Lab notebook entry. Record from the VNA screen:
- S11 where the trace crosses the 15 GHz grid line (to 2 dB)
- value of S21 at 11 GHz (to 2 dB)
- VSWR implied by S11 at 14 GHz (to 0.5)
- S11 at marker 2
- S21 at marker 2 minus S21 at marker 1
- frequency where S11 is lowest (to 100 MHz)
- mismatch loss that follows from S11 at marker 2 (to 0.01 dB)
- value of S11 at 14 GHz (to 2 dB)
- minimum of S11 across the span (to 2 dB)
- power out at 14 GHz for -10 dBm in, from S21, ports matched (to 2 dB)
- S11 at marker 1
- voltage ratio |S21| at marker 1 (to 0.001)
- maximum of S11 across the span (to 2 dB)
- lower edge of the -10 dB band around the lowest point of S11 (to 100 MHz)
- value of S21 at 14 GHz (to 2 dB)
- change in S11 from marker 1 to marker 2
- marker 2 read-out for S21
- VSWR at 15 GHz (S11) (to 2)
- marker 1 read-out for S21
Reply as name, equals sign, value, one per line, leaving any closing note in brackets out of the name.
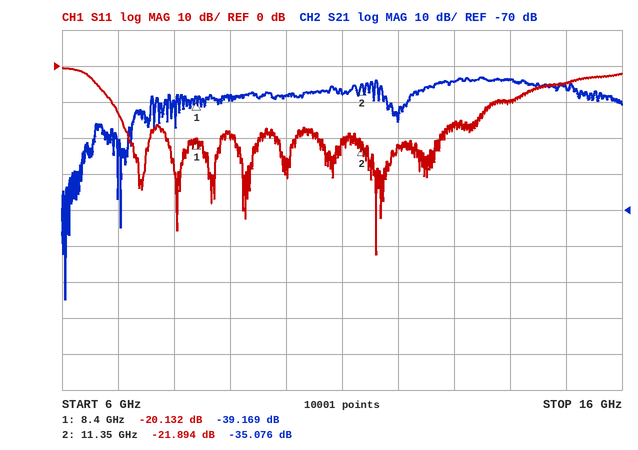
S11 where the trace crosses the 15 GHz grid line = -4 dB
value of S21 at 11 GHz = -38 dB
VSWR implied by S11 at 14 GHz = 2.0
S11 at marker 2 = -21.894 dB
S21 at marker 2 minus S21 at marker 1 = 4.093 dB
frequency where S11 is lowest = 11.6 GHz
mismatch loss that follows from S11 at marker 2 = 0.03 dB
value of S11 at 14 GHz = -10 dB
minimum of S11 across the span = -52 dB
power out at 14 GHz for -10 dBm in, from S21, ports matched = -44 dBm
S11 at marker 1 = -20.132 dB
voltage ratio |S21| at marker 1 = 0.011
maximum of S11 across the span = 0 dB
lower edge of the -10 dB band around the lowest point of S11 = 6.9 GHz
value of S21 at 14 GHz = -34 dB
change in S11 from marker 1 to marker 2 = -1.762 dB
marker 2 read-out for S21 = -35.076 dB
VSWR at 15 GHz (S11) = 4
marker 1 read-out for S21 = -39.169 dB
